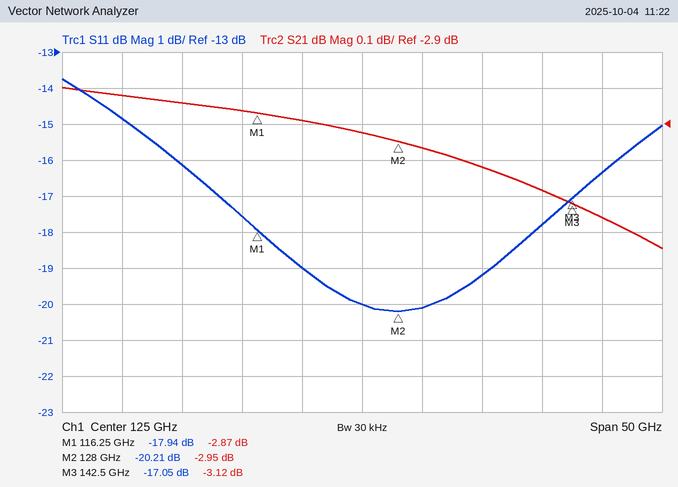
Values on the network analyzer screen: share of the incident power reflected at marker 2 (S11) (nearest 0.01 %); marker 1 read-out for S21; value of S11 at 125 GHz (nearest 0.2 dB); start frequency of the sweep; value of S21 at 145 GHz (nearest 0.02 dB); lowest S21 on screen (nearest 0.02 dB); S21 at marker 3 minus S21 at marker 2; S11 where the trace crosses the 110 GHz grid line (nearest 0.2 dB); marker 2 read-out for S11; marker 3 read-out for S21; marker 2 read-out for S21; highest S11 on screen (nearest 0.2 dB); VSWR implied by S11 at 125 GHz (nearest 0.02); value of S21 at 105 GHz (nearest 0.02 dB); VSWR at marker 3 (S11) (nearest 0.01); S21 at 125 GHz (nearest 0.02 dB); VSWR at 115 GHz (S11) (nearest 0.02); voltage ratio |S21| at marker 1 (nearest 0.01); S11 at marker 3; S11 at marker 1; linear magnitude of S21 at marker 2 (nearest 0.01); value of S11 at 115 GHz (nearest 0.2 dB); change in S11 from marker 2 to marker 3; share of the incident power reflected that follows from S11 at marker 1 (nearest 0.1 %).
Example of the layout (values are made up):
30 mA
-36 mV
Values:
0.95 %
-2.87 dB
-20.0 dB
100 GHz
-3.16 dB
-3.24 dB
-0.17 dB
-16.2 dB
-20.21 dB
-3.12 dB
-2.95 dB
-13.8 dB
1.22
-2.82 dB
1.33
-2.92 dB
1.30
0.72
-17.05 dB
-17.94 dB
0.71
-17.6 dB
3.16 dB
1.6 %
